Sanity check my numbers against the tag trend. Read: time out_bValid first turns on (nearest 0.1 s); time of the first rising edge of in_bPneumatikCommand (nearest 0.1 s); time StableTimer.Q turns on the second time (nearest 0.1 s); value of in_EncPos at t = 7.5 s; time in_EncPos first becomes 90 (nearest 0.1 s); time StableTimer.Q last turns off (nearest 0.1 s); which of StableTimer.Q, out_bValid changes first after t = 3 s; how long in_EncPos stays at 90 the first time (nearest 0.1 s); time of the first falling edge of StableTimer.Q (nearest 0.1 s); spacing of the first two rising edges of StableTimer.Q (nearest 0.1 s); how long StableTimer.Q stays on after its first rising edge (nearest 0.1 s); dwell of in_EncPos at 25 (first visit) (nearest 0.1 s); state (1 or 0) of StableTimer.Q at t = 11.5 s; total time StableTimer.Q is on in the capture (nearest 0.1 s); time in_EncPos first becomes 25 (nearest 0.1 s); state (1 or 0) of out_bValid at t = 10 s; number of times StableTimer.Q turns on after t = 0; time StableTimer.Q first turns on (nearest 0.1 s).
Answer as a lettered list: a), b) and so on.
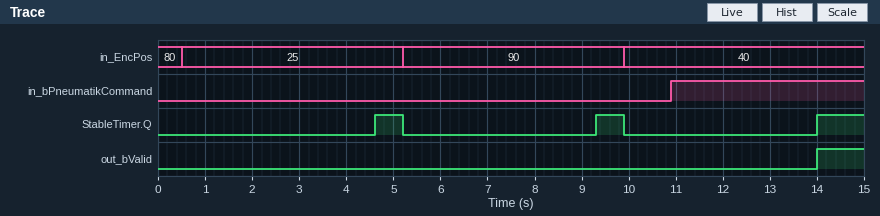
a) 14.0 s
b) 10.9 s
c) 9.3 s
d) 90
e) 5.2 s
f) 9.9 s
g) StableTimer.Q
h) 4.7 s
i) 5.2 s
j) 4.7 s
k) 0.6 s
l) 4.7 s
m) 0
n) 2.2 s
o) 0.5 s
p) 0
q) 3
r) 4.6 s
